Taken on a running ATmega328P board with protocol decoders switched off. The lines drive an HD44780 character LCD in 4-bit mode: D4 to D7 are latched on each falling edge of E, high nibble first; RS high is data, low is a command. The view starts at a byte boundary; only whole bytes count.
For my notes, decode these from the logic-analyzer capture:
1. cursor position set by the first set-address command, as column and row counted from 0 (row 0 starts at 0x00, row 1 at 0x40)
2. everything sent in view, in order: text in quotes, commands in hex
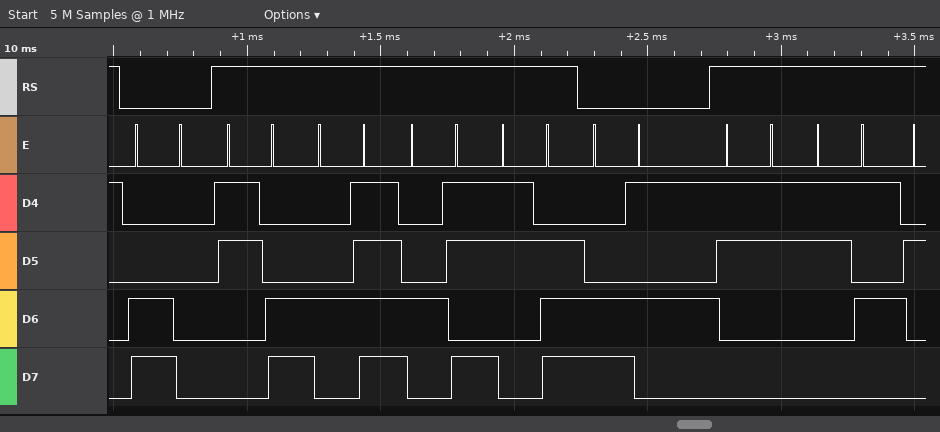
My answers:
column 0, row 1
0xC0 "<OK>" 0xC5 "35"
